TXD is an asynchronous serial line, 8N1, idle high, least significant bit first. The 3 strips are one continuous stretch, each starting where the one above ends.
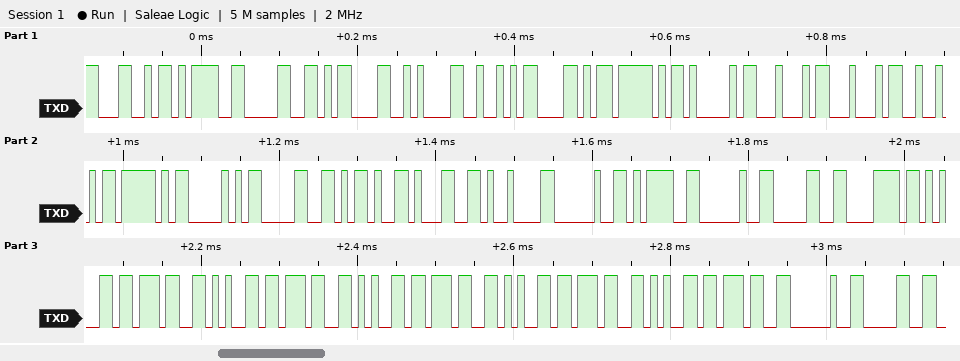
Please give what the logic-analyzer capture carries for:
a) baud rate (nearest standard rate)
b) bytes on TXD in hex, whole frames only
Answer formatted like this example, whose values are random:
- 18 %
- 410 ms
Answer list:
- 115200 baud
- 4C 3D 30 0D 0A 52 58 5F 41 44 44 52 5F 50 30 2D 31 09 20 3D 20 30 78 65 37 65 37 65 37 65 37 65 37 20 30
